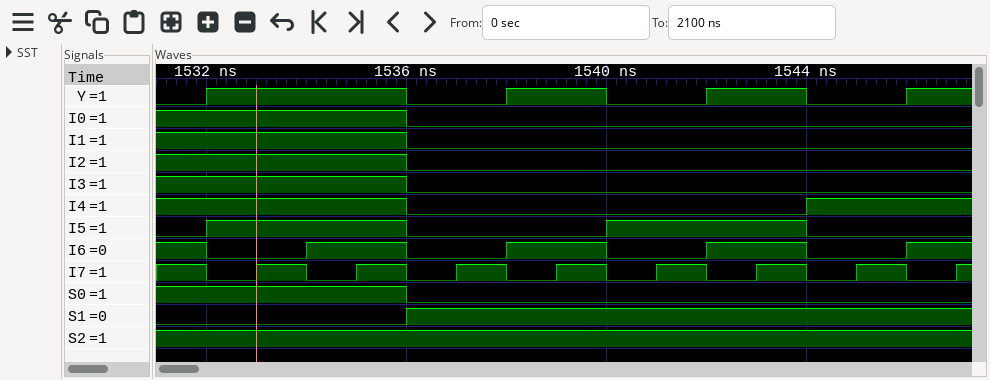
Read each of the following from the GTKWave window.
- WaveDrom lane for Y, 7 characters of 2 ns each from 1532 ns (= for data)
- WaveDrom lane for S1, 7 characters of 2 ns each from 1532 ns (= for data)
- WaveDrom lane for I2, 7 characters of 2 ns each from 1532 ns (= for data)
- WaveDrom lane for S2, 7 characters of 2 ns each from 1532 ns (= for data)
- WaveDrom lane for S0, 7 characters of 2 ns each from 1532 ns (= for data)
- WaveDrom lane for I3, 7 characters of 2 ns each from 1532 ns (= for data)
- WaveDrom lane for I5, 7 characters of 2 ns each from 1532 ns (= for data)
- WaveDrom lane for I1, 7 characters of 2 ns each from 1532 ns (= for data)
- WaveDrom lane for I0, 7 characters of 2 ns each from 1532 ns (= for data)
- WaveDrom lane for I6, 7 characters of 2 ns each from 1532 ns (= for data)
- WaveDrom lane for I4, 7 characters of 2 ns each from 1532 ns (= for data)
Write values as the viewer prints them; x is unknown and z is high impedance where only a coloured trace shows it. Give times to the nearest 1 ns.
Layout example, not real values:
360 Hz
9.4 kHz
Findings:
{name: 'Y', wave: '1.01010'}
{name: 'S1', wave: '0.1....'}
{name: 'I2', wave: '1.0....'}
{name: 'S2', wave: '1......'}
{name: 'S0', wave: '1.0....'}
{name: 'I3', wave: '1.0....'}
{name: 'I5', wave: '1.0.1.0'}
{name: 'I1', wave: '1.0....'}
{name: 'I0', wave: '1.0....'}
{name: 'I6', wave: '0101010'}
{name: 'I4', wave: '1.0...1'}
